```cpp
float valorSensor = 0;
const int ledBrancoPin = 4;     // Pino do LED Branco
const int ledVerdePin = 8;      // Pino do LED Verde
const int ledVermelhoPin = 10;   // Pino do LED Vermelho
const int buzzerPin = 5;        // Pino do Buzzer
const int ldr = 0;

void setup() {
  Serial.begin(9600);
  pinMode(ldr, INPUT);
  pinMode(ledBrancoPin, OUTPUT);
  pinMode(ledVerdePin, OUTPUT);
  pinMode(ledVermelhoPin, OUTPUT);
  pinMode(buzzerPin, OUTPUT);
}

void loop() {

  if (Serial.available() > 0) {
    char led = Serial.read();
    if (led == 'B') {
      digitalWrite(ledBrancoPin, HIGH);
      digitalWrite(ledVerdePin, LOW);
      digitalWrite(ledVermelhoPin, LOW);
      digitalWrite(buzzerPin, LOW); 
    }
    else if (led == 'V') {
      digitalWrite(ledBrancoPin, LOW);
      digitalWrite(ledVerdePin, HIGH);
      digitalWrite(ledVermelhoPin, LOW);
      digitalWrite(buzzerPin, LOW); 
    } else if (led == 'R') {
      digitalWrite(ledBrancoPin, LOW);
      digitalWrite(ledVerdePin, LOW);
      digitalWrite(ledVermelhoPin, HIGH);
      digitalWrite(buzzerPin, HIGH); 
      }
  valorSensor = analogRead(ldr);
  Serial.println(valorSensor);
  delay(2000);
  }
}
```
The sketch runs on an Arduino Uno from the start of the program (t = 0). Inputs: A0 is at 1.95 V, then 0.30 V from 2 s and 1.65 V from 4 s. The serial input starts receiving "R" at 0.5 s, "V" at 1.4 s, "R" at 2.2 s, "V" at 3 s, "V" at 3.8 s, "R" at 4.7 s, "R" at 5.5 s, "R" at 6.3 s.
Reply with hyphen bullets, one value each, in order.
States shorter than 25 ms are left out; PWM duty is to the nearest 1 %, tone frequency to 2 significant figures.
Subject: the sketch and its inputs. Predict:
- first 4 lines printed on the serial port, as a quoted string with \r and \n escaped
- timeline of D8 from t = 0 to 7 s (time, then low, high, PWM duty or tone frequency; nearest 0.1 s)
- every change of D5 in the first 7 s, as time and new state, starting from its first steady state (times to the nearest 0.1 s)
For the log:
- "399.00\r\n61.00\r\n337.00\r\n337.00\r\n"
- 0 s low; 2.5 s high; 4.5 s low; 6.5 s high
- 0 s low; 0.5 s high; 2.5 s low; 4.5 s high; 6.5 s low
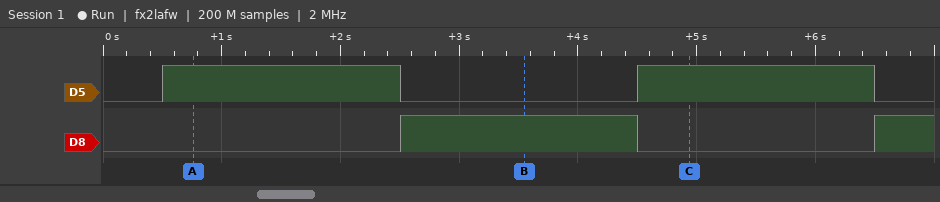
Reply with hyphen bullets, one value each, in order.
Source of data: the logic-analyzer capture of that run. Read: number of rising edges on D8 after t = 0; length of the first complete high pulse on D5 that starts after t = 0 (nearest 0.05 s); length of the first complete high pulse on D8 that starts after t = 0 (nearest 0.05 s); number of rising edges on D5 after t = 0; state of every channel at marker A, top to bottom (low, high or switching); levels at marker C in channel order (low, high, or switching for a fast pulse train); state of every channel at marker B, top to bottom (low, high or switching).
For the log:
- 2
- 2.00 s
- 2.00 s
- 2
- D5 high, D8 low
- D5 high, D8 low
- D5 low, D8 high
